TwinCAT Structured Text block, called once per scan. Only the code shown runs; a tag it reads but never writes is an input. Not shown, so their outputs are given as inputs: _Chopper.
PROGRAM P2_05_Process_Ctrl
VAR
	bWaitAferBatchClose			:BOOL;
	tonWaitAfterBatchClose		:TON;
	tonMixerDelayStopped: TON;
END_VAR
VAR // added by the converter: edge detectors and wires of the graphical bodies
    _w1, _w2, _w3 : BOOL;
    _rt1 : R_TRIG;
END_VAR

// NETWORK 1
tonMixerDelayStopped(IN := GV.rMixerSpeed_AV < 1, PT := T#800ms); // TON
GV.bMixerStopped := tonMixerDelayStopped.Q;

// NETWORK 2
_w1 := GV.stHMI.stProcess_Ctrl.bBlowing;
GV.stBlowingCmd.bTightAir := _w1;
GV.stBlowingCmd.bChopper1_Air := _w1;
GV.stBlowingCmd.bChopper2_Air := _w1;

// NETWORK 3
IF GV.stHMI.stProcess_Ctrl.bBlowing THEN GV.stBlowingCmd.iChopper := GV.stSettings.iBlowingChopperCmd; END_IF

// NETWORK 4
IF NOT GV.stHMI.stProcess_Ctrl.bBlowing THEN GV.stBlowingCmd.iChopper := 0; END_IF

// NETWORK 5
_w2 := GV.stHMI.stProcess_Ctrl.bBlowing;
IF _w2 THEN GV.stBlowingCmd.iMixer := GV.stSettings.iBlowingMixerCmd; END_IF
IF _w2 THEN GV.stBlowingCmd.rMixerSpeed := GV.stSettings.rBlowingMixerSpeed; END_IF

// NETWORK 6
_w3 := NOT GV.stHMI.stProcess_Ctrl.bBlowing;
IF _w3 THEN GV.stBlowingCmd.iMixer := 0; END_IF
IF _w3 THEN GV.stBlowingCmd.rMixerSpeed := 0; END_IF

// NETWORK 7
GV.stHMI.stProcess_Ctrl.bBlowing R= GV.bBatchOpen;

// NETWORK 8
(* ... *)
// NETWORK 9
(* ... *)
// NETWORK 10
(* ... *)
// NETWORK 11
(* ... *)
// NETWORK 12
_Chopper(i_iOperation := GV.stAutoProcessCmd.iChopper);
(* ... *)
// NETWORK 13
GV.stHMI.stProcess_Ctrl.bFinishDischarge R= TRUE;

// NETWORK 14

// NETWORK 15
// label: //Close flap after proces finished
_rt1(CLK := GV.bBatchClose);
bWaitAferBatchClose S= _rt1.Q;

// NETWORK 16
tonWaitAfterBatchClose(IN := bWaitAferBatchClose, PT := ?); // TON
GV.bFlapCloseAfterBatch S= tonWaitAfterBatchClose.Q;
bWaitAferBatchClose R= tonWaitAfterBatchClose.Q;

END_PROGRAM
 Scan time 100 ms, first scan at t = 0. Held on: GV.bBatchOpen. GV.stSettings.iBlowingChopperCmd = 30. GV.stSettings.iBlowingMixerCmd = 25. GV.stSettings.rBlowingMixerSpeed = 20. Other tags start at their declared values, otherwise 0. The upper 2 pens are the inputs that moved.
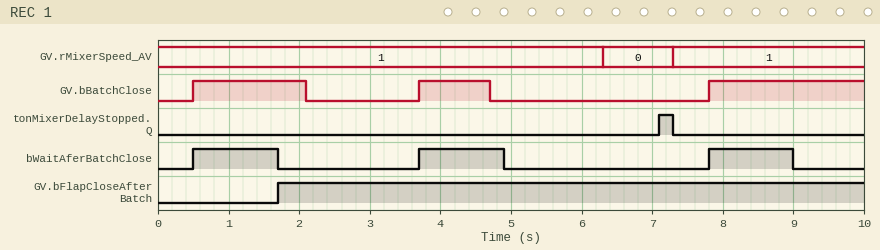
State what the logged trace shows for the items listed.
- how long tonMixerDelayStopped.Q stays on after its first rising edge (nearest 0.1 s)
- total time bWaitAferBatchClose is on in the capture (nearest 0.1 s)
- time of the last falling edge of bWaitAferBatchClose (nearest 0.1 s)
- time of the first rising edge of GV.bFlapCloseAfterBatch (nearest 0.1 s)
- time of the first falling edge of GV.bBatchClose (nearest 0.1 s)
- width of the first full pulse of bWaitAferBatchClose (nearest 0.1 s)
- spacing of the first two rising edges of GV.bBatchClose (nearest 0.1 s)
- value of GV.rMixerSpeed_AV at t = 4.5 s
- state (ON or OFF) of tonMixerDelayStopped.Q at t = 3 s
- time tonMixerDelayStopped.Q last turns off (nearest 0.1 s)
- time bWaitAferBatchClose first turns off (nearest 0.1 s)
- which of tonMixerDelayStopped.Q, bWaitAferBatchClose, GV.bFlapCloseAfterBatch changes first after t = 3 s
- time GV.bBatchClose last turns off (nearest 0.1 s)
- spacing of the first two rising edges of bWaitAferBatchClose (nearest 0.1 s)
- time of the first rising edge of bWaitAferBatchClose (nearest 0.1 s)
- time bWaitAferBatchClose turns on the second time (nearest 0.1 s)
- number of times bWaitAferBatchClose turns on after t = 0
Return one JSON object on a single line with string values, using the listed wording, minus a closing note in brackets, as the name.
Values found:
{"how long tonMixerDelayStopped.Q stays on after its first rising edge": "0.2 s", "total time bWaitAferBatchClose is on in the capture": "3.6 s", "time of the last falling edge of bWaitAferBatchClose": "9.0 s", "time of the first rising edge of GV.bFlapCloseAfterBatch": "1.7 s", "time of the first falling edge of GV.bBatchClose": "2.1 s", "width of the first full pulse of bWaitAferBatchClose": "1.2 s", "spacing of the first two rising edges of GV.bBatchClose": "3.2 s", "value of GV.rMixerSpeed_AV at t = 4.5 s": "1", "state (ON or OFF) of tonMixerDelayStopped.Q at t = 3 s": "OFF", "time tonMixerDelayStopped.Q last turns off": "7.3 s", "time bWaitAferBatchClose first turns off": "1.7 s", "which of tonMixerDelayStopped.Q, bWaitAferBatchClose, GV.bFlapCloseAfterBatch changes first after t = 3 s": "bWaitAferBatchClose", "time GV.bBatchClose last turns off": "4.7 s", "spacing of the first two rising edges of bWaitAferBatchClose": "3.2 s", "time of the first rising edge of bWaitAferBatchClose": "0.5 s", "time bWaitAferBatchClose turns on the second time": "3.7 s", "number of times bWaitAferBatchClose turns on after t = 0": "3"}
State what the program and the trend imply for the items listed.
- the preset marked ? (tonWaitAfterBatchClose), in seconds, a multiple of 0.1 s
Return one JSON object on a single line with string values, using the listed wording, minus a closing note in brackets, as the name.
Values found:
{"the preset marked ? (tonWaitAfterBatchClose), in seconds, a multiple of 0.1 s": "1.2 s"}
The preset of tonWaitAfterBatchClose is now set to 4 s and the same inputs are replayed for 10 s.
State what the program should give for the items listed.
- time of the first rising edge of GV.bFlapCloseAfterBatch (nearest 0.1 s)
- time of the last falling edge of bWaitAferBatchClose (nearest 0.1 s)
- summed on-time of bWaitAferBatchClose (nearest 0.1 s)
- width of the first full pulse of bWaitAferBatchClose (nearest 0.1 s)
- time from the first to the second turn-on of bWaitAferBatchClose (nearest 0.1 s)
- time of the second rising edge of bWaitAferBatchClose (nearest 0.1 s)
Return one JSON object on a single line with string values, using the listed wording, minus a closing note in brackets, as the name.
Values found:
{"time of the first rising edge of GV.bFlapCloseAfterBatch": "4.5 s", "time of the last falling edge of bWaitAferBatchClose": "4.5 s", "summed on-time of bWaitAferBatchClose": "6.2 s", "width of the first full pulse of bWaitAferBatchClose": "4.0 s", "time from the first to the second turn-on of bWaitAferBatchClose": "7.3 s", "time of the second rising edge of bWaitAferBatchClose": "7.8 s"}
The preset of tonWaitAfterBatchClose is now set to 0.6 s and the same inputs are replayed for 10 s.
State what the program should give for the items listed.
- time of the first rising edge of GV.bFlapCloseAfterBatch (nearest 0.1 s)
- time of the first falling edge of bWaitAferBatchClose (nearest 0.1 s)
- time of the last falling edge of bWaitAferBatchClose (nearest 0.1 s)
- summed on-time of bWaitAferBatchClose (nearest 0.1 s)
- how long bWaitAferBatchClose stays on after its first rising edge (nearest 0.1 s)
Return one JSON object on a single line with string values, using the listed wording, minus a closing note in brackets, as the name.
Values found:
{"time of the first rising edge of GV.bFlapCloseAfterBatch": "1.1 s", "time of the first falling edge of bWaitAferBatchClose": "1.1 s", "time of the last falling edge of bWaitAferBatchClose": "8.4 s", "summed on-time of bWaitAferBatchClose": "1.8 s", "how long bWaitAferBatchClose stays on after its first rising edge": "0.6 s"}
